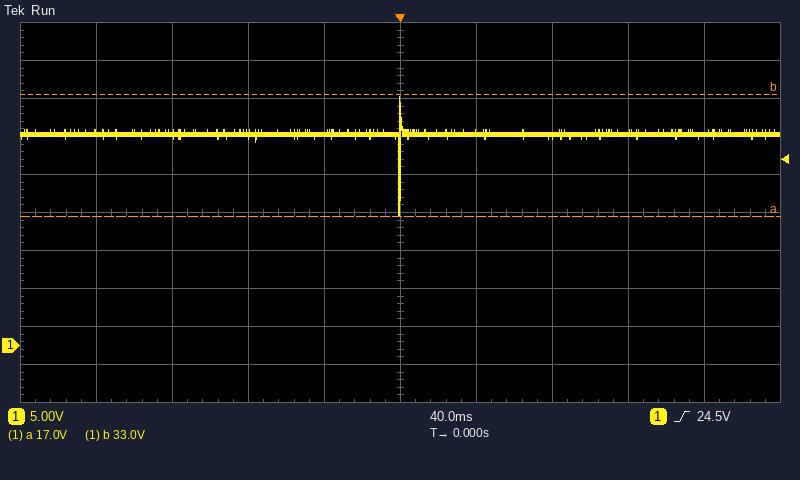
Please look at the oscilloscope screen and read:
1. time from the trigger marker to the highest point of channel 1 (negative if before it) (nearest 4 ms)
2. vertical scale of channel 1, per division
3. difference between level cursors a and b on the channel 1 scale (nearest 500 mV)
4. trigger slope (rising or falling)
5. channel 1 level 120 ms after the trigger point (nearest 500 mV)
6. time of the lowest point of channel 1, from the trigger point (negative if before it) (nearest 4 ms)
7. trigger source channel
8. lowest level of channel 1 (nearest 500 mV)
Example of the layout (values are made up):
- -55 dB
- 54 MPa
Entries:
- 0 ms
- 5 V
- 16.0 V
- rising
- 28.0 V
- 0 ms
- channel 1
- 17.0 V
